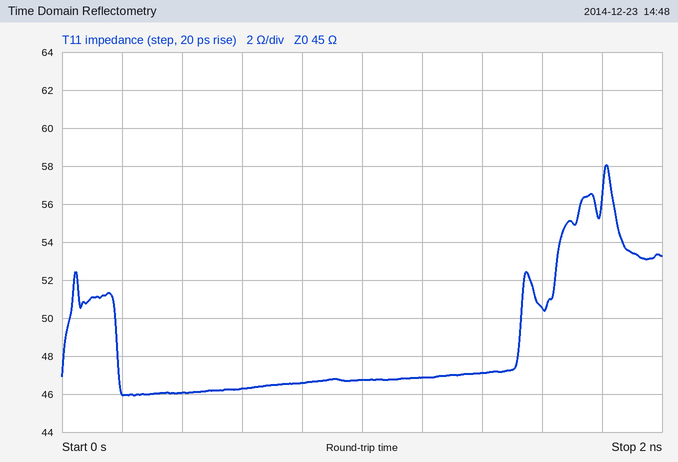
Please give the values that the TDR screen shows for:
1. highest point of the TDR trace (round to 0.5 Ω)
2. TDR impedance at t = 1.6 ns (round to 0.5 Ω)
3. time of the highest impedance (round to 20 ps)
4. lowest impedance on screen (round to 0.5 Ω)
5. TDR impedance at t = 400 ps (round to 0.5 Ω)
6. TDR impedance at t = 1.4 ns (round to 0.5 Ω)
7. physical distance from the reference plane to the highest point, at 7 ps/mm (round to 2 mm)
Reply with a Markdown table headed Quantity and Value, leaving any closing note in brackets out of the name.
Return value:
| Quantity | Value |
|---|---|
| highest point of the TDR trace | 58.0 Ω |
| TDR impedance at t = 1.6 ns | 50.5 Ω |
| time of the highest impedance | 1.82 ns |
| lowest impedance on screen | 46.0 Ω |
| TDR impedance at t = 400 ps | 46.0 Ω |
| TDR impedance at t = 1.4 ns | 47.0 Ω |
| physical distance from the reference plane to the highest point, at 7 ps/mm | 130 mm |
